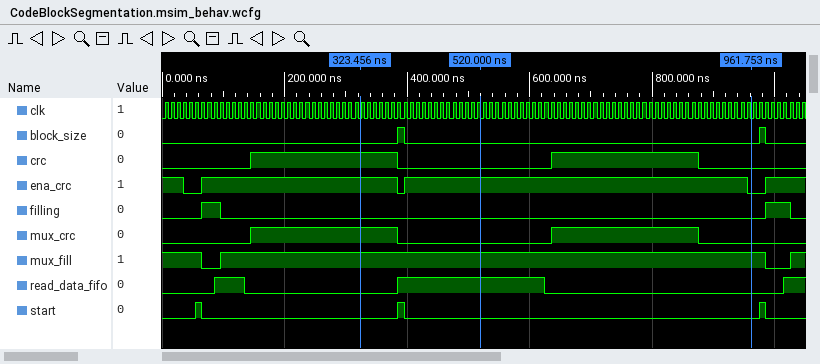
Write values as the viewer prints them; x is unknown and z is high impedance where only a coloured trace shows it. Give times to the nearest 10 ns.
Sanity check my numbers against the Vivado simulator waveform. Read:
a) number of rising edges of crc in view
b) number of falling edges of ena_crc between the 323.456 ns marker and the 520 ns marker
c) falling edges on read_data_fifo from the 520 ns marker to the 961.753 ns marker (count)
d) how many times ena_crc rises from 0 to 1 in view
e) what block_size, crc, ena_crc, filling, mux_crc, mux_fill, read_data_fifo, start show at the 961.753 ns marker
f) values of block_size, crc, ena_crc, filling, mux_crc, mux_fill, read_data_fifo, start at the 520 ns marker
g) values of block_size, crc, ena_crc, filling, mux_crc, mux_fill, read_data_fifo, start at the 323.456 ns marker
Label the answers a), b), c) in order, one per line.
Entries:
a) 2
b) 1
c) 1
d) 3
e) block_size=0, crc=0, ena_crc=0, filling=0, mux_crc=0, mux_fill=1, read_data_fifo=0, start=0
f) block_size=0, crc=0, ena_crc=1, filling=0, mux_crc=0, mux_fill=1, read_data_fifo=1, start=0
g) block_size=0, crc=1, ena_crc=1, filling=0, mux_crc=1, mux_fill=1, read_data_fifo=0, start=0
